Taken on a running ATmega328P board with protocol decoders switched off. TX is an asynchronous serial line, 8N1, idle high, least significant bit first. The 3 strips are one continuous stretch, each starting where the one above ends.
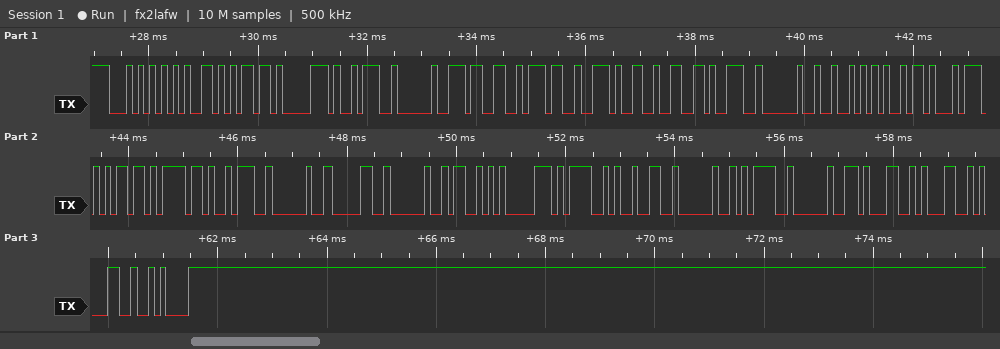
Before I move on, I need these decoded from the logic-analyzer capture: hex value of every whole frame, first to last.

54 65 6D 70 3A 20 33 37 2E 32 39 20 52 69 74 6D 6F 3A 20 30 20 53 70 4F 32 20 3D 20 31 31 31 0A
